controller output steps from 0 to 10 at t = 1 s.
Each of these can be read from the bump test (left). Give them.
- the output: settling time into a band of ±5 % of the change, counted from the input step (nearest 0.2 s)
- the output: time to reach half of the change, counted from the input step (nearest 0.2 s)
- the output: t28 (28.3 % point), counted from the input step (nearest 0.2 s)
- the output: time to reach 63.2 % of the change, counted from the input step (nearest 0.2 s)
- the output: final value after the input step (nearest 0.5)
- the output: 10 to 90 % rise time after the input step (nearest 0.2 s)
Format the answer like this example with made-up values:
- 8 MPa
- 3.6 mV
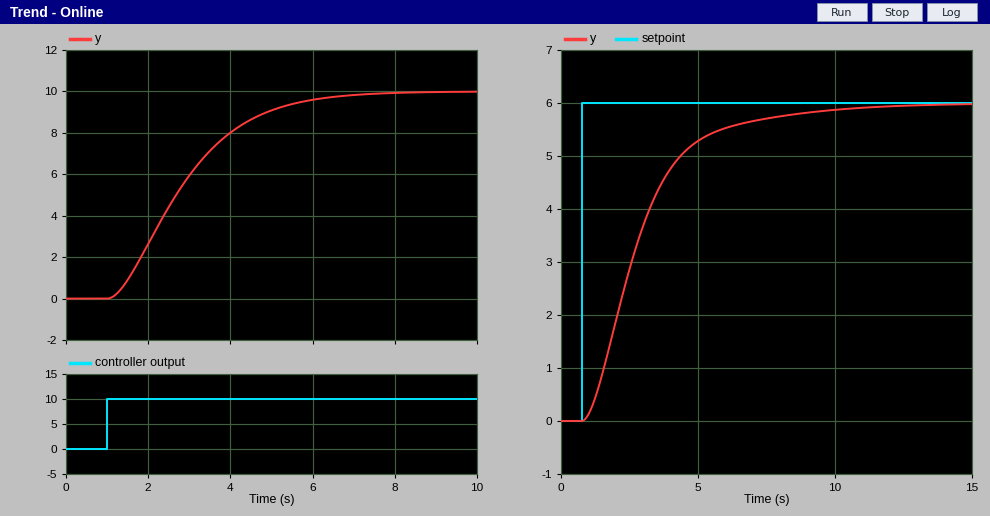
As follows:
- 4.8 s
- 1.6 s
- 1.0 s
- 2.2 s
- 10.0
- 3.4 s
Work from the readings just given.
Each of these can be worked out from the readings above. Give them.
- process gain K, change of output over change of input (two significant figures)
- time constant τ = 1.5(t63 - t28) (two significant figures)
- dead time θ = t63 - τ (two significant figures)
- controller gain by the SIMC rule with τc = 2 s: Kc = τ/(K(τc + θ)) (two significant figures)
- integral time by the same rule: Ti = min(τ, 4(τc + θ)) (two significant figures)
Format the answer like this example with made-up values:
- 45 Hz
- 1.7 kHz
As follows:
- 1.0
- 1.8 s
- 0.40 s
- 0.75
- 1.8 s
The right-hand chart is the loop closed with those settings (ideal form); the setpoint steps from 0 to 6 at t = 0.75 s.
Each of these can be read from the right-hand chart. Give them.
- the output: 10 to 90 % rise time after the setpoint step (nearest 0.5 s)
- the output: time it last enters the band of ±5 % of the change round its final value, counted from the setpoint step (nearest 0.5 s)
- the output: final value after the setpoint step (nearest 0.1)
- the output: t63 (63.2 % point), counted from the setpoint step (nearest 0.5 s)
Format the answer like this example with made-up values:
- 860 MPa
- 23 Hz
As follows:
- 4.0 s
- 6.5 s
- 6.0
- 2.5 s
